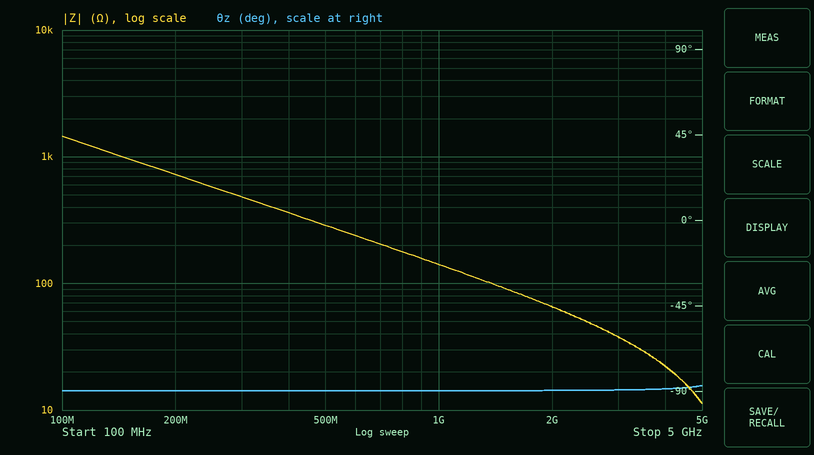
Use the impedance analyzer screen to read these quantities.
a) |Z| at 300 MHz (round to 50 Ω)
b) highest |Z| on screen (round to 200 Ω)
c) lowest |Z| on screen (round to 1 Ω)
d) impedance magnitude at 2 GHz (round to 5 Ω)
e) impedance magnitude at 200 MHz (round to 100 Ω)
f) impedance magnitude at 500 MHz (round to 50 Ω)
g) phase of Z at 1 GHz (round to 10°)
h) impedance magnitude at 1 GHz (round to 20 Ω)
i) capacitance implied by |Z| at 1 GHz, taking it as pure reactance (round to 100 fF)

500 Ω
1.4 kΩ
11 Ω
65 Ω
700 Ω
300 Ω
-90°
140 Ω
1.1 pF
